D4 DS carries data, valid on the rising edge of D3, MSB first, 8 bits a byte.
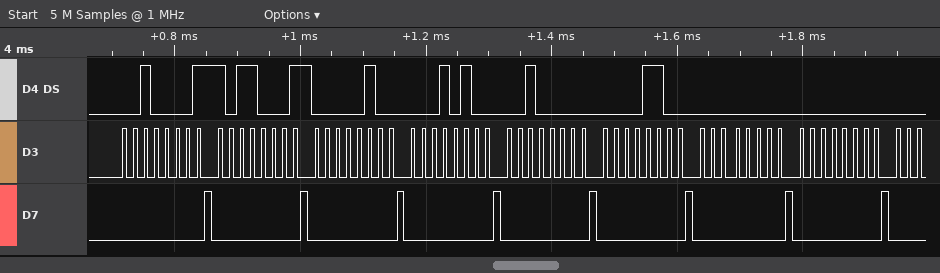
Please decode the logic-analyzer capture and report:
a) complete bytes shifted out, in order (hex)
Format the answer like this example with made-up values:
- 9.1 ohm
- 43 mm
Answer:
- 21 B1 04 14 20 0C 00 00
